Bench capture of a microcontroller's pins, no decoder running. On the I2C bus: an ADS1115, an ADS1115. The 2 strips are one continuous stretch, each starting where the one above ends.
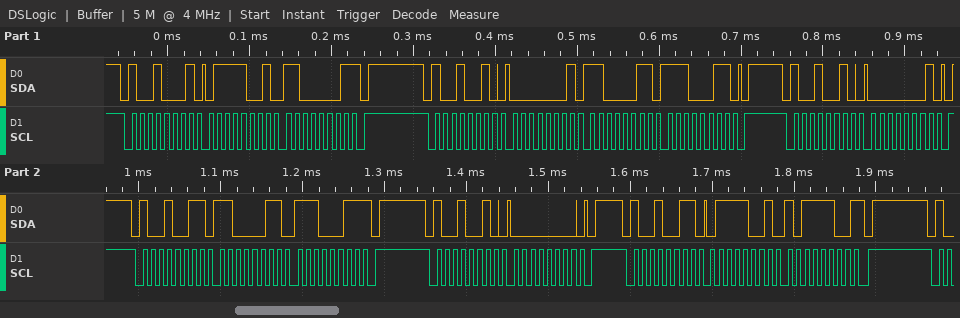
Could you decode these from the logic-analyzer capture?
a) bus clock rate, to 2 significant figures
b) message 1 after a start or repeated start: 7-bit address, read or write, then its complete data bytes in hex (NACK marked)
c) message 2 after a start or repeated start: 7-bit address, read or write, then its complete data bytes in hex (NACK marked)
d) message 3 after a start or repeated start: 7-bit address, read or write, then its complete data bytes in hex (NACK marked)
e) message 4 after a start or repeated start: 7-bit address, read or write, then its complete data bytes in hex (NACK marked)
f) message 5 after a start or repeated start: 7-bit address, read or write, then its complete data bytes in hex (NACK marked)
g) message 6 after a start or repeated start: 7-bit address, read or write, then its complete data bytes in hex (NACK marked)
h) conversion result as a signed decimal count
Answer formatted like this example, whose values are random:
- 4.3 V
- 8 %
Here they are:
- 100 kHz
- 0x48 read: 79 C1 NACK
- 0x49 write: 01 C3 E3
- 0x49 write: 01
- 0x49 read: C3 E3 NACK
- 0x49 write: 00
- 0x49 read: 79 BC NACK
- 31164
